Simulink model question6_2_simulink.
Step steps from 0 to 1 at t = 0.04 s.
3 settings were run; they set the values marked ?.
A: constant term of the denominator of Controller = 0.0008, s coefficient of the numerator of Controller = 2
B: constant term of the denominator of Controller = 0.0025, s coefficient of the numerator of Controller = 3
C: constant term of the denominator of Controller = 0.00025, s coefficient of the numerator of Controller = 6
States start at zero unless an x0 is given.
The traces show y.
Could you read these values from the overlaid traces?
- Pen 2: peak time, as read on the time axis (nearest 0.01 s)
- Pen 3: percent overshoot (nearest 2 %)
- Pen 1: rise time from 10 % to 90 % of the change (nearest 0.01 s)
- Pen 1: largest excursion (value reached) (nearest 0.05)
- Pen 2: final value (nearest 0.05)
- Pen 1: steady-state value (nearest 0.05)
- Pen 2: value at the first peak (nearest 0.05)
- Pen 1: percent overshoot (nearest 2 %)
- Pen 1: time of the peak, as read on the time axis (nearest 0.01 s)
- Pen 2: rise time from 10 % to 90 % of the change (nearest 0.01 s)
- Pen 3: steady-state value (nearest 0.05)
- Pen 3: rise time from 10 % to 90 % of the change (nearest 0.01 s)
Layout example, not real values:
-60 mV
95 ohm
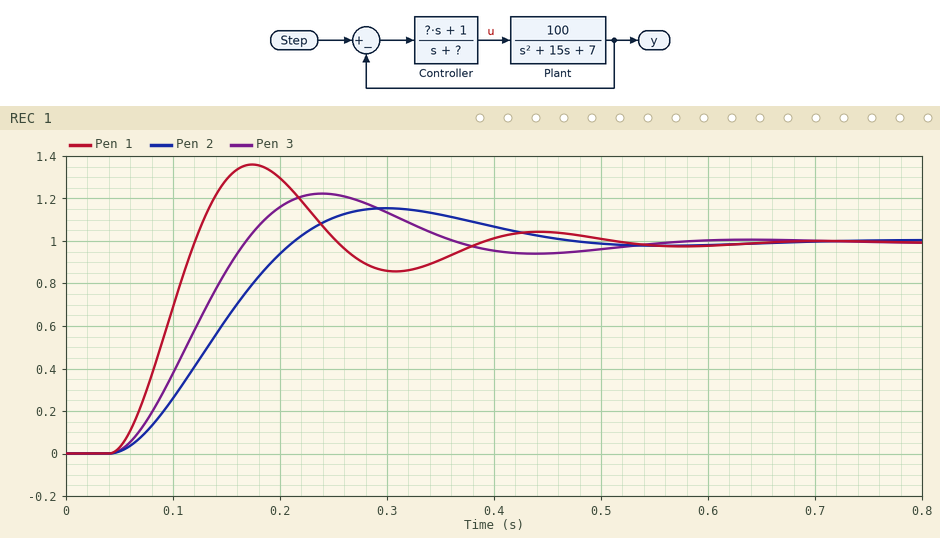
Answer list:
0.30 s
22 %
0.05 s
1.35
1.00
1.00
1.15
36 %
0.17 s
0.12 s
1.00
0.09 s
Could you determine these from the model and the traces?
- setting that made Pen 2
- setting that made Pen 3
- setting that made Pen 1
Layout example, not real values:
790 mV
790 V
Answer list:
A
B
C
